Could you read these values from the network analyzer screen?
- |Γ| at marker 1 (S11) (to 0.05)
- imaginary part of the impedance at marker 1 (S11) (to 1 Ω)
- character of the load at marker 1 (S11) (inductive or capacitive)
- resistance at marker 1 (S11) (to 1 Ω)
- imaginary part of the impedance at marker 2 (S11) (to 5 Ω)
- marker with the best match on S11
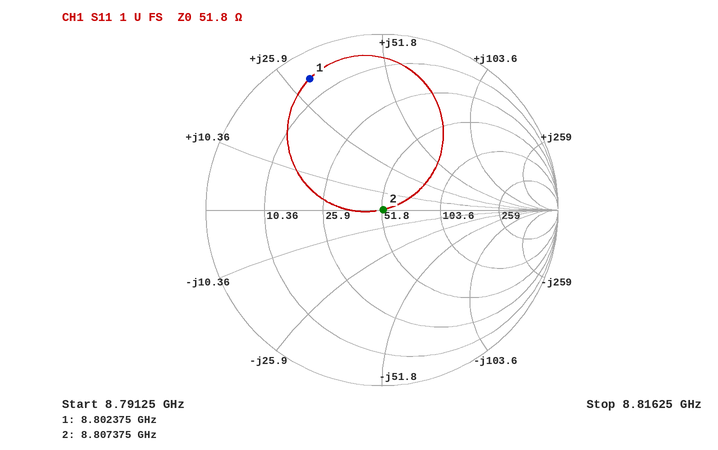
0.85
+30 Ω
inductive
6 Ω
0 Ω
marker 2
